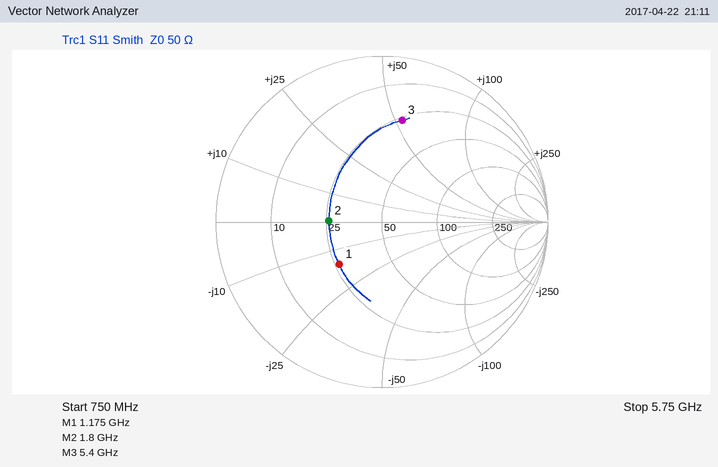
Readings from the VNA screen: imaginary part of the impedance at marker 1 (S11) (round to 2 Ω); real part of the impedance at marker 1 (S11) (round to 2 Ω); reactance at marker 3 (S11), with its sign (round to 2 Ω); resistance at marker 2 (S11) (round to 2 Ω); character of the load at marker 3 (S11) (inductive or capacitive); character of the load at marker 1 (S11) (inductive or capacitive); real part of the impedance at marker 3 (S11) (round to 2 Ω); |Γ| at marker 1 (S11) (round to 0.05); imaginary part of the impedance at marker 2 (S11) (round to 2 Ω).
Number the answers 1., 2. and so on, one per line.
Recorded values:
1. -16 Ω
2. 26 Ω
3. +54 Ω
4. 26 Ω
5. inductive
6. capacitive
7. 26 Ω
8. 0.35
9. 0 Ω
